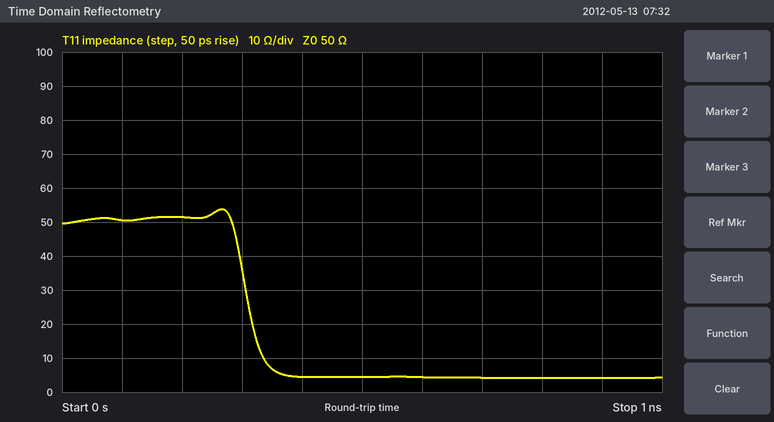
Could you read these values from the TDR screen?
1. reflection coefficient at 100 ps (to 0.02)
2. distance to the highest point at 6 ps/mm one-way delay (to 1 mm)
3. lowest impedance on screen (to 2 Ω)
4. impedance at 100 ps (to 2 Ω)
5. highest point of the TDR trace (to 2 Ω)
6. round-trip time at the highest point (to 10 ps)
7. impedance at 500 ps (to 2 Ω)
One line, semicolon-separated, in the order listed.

0.00; 22 mm; 4 Ω; 50 Ω; 54 Ω; 270 ps; 4 Ω
